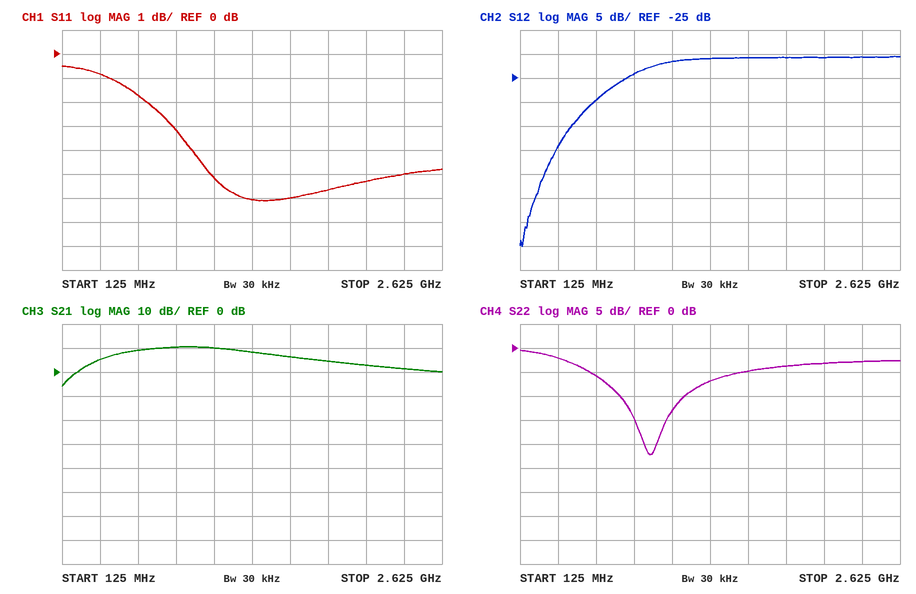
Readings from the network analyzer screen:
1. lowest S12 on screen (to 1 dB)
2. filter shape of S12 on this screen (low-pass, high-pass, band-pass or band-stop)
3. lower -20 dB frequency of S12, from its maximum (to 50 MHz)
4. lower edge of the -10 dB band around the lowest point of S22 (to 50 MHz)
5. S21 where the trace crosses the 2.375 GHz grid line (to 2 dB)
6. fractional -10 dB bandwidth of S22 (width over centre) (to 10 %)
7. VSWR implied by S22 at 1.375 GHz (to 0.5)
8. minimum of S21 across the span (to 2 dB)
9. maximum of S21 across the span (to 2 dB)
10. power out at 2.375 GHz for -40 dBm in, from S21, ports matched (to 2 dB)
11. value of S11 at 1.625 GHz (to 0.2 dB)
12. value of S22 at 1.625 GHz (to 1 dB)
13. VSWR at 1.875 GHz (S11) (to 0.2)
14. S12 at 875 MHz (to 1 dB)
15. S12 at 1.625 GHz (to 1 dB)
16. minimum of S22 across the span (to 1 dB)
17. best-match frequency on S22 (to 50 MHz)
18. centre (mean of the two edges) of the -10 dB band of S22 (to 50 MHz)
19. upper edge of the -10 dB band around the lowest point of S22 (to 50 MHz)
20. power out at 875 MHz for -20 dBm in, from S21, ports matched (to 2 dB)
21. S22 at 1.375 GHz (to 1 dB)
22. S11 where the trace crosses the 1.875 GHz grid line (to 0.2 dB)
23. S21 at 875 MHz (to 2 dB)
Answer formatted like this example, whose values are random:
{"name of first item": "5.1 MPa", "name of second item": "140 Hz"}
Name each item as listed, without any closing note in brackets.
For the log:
{"lowest S12 on screen": "-60 dB", "filter shape of S12 on this screen": "high-pass", "lower -20 dB frequency of S12, from its maximum": "350 MHz", "lower edge of the -10 dB band around the lowest point of S22": "800 MHz", "S21 where the trace crosses the 2.375 GHz grid line": "2 dB", "fractional -10 dB bandwidth of S22 (width over centre)": "40 %", "VSWR implied by S22 at 1.375 GHz": "2.5", "minimum of S21 across the span": "-6 dB", "maximum of S21 across the span": "10 dB", "power out at 2.375 GHz for -40 dBm in, from S21, ports matched": "-38 dBm", "value of S11 at 1.625 GHz": "-6.0 dB", "value of S22 at 1.625 GHz": "-5 dB", "VSWR at 1.875 GHz (S11)": "3.2", "S12 at 875 MHz": "-24 dB", "S12 at 1.625 GHz": "-21 dB", "minimum of S22 across the span": "-22 dB", "best-match frequency on S22": "1.00 GHz", "centre (mean of the two edges) of the -10 dB band of S22": "1.00 GHz", "upper edge of the -10 dB band around the lowest point of S22": "1.20 GHz", "power out at 875 MHz for -20 dBm in, from S21, ports matched": "-10 dBm", "S22 at 1.375 GHz": "-7 dB", "S11 where the trace crosses the 1.875 GHz grid line": "-5.6 dB", "S21 at 875 MHz": "10 dB"}
